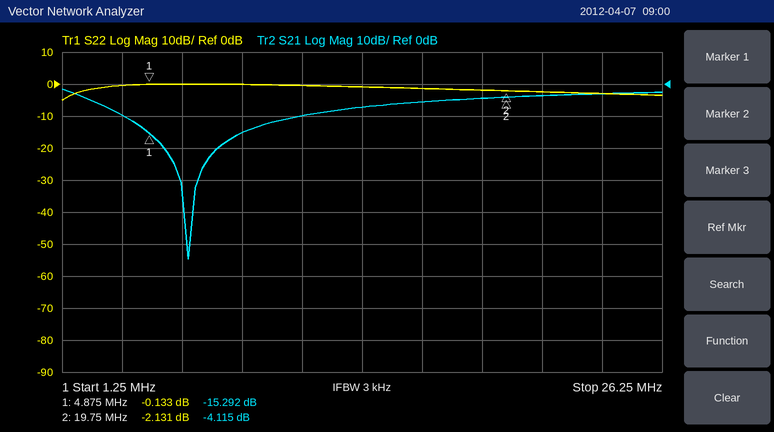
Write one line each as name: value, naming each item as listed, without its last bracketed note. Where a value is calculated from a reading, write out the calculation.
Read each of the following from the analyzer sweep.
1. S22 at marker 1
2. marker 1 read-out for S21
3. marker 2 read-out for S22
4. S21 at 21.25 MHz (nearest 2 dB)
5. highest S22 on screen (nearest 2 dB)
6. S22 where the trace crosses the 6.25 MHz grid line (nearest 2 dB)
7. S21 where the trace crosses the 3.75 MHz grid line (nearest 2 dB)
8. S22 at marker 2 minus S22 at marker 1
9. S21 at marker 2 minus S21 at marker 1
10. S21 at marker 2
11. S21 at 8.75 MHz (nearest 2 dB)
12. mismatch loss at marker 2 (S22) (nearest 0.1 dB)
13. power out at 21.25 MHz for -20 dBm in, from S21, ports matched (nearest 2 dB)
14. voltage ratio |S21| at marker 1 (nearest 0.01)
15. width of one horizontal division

S22 at marker 1: -0.133 dB
marker 1 read-out for S21: -15.292 dB
marker 2 read-out for S22: -2.131 dB
S21 at 21.25 MHz: -4 dB
highest S22 on screen: 0 dB
S22 where the trace crosses the 6.25 MHz grid line: 0 dB
S21 where the trace crosses the 3.75 MHz grid line: -10 dB
S22 at marker 2 minus S22 at marker 1: -2.131 − (-0.133) = -1.998 dB
S21 at marker 2 minus S21 at marker 1: -4.115 − (-15.292) = 11.177 dB
S21 at marker 2: -4.115 dB
S21 at 8.75 MHz: -16 dB
mismatch loss at marker 2 (S22): −10 log10(1 − 10^(-2.131/10)) ≈ 4.1 dB
power out at 21.25 MHz for -20 dBm in, from S21, ports matched: -20 dBm + (-4 dB) = -24 dBm
voltage ratio |S21| at marker 1: 10^(-15.292/20) ≈ 0.17
width of one horizontal division: 2.5 MHz
